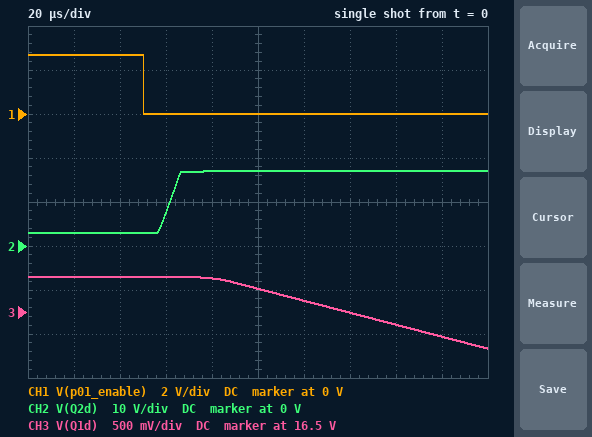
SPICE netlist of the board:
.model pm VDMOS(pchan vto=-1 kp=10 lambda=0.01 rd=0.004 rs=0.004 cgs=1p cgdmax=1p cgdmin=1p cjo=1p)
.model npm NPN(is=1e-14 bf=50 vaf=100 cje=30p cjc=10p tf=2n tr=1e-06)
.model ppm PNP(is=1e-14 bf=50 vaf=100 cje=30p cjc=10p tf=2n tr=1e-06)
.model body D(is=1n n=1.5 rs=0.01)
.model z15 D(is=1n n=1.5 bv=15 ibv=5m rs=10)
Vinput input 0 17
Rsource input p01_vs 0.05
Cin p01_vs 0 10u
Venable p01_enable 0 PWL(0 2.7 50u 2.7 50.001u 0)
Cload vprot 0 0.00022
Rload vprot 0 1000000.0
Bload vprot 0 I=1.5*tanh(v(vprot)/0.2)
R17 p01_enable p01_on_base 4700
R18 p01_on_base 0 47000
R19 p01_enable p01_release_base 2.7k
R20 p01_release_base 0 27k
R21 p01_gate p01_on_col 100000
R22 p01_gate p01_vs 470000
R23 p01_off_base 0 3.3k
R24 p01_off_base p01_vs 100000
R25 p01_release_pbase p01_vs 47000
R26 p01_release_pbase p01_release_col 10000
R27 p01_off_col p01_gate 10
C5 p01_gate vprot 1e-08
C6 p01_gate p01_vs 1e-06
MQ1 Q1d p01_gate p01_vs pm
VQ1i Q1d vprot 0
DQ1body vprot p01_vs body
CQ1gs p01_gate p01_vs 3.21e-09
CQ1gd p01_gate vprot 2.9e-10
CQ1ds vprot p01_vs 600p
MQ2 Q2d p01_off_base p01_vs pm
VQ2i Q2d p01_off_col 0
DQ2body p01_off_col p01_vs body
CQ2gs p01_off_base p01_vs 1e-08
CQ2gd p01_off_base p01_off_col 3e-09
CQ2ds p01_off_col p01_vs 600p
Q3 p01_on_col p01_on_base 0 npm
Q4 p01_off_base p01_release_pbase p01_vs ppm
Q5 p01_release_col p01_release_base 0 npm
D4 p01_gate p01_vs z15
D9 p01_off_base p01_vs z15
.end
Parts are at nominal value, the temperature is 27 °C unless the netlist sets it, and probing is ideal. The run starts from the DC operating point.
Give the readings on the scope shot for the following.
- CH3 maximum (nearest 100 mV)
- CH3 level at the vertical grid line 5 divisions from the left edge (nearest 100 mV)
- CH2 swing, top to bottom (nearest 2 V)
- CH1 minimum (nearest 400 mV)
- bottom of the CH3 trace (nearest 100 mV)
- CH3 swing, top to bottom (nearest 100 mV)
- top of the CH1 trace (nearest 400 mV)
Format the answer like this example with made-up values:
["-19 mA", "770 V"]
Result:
["16.9 V", "16.8 V", "14 V", "0 V", "16.1 V", "800 mV", "2.8 V"]
